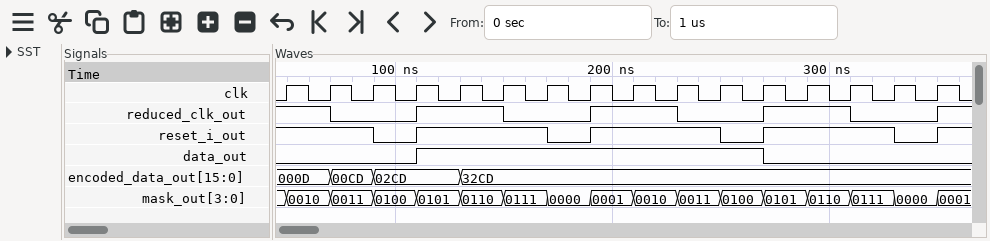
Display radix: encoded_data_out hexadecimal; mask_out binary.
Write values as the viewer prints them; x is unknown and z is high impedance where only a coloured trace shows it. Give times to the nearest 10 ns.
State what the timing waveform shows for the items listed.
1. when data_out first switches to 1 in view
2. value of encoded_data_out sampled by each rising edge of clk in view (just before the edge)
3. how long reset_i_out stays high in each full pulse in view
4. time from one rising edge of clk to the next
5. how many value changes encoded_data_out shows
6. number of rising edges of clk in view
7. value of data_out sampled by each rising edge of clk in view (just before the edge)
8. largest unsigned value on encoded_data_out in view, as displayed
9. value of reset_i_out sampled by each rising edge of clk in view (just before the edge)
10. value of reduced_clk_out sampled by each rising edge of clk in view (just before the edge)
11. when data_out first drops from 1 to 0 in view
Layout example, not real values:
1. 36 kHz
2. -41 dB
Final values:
1. 110 ns
2. 000D, 000D, 00CD, 02CD, 02CD, 32CD, 32CD, 32CD, 32CD, 32CD, 32CD, 32CD, 32CD, 32CD, 32CD, 32CD
3. 60 ns, 60 ns, 60 ns
4. 20 ns
5. 3
6. 16
7. 0 0 0 0 1 1 1 1 1 1 1 1 0 0 0 0
8. 32CD
9. 1 1 1 0 1 1 1 0 1 1 1 0 1 1 1 0
10. 1 1 0 0 1 1 0 0 1 1 0 0 1 1 0 0
11. 270 ns
